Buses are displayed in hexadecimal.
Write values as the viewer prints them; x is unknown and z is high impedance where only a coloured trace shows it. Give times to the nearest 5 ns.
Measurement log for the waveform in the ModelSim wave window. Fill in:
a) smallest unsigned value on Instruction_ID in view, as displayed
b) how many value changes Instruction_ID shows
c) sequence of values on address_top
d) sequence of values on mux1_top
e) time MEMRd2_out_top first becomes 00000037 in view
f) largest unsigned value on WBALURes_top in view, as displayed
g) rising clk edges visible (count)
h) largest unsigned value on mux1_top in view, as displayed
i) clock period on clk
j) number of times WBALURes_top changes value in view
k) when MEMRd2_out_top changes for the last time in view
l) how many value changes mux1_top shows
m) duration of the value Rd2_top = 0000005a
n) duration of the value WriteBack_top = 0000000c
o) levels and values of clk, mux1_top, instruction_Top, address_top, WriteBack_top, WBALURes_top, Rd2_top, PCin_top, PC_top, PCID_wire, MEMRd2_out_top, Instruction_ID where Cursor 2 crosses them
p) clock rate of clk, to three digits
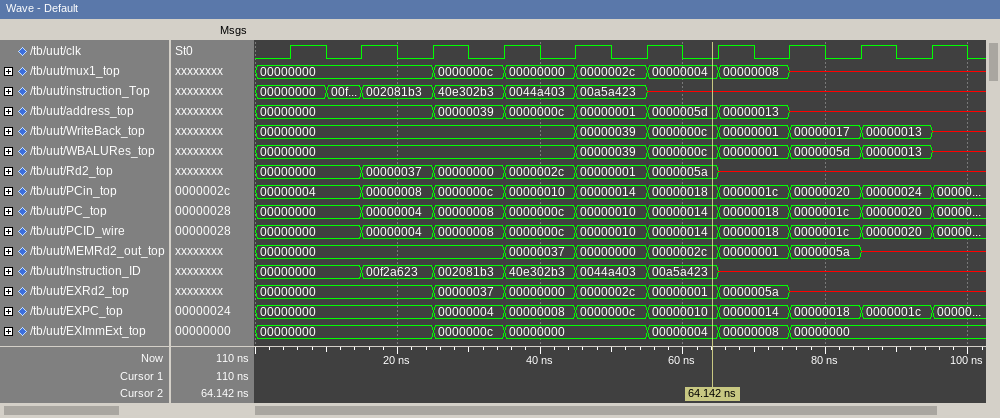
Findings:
00000000
6
00000000, 00000039, 0000000c, 00000001, 0000005d, 00000013, x
00000000, 0000000c, 00000000, 0000002c, 00000004, 00000008, x
35 ns
0000005d
10
0000002c
10 ns
6
85 ns
6
10 ns
10 ns
clk=0, mux1_top=00000004, instruction_Top=x, address_top=0000005d, WriteBack_top=0000000c, WBALURes_top=0000000c, Rd2_top=0000005a, PCin_top=00000018, PC_top=00000014, PCID_wire=00000014, MEMRd2_out_top=0000002c, Instruction_ID=00a5a423
100 MHz
